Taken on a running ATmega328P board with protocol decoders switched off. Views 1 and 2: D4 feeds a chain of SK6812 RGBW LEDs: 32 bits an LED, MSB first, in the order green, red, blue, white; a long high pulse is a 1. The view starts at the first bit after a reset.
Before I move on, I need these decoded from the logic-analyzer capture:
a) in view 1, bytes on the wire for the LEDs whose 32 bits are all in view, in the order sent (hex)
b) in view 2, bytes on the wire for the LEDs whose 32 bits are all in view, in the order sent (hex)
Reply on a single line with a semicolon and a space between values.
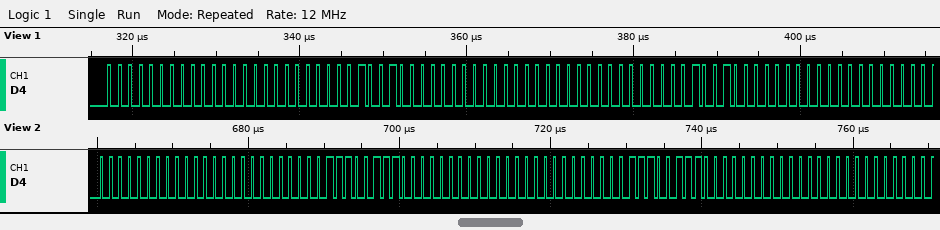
00 00 00 90 00 00 00 90; 00 00 00 E7 00 00 00 E7
